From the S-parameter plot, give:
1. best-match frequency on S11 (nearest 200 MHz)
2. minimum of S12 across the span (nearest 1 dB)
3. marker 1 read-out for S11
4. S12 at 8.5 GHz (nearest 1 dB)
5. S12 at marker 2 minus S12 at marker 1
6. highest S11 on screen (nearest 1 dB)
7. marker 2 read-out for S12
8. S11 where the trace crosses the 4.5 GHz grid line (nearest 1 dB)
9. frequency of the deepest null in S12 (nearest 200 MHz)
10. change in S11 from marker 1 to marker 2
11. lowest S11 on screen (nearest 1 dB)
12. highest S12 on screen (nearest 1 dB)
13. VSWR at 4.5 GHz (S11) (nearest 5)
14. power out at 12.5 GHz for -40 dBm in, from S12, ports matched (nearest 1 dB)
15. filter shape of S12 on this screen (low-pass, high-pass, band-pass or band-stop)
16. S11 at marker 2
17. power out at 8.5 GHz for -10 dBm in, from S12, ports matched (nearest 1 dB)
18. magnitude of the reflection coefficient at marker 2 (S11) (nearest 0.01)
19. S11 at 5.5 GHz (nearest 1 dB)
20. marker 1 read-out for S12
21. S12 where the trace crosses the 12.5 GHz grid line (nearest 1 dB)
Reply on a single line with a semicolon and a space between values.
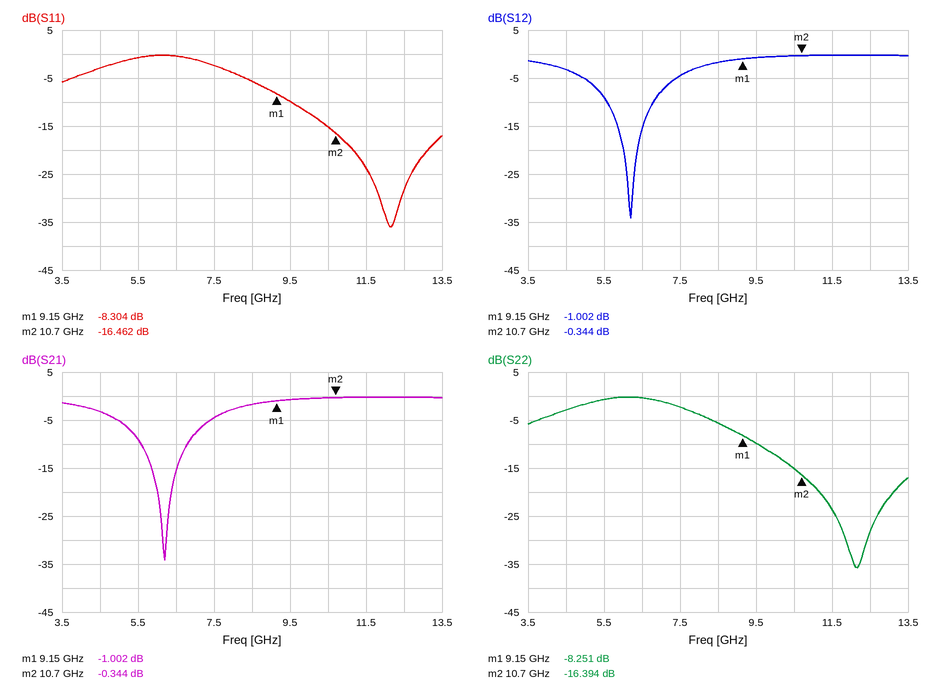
12.2 GHz; -34 dB; -8.304 dB; -2 dB; 0.658 dB; 0 dB; -0.344 dB; -3 dB; 6.2 GHz; -8.158 dB; -36 dB; 0 dB; 5; -40 dBm; band-stop; -16.462 dB; -12 dBm; 0.15; -1 dB; -1.002 dB; 0 dB
